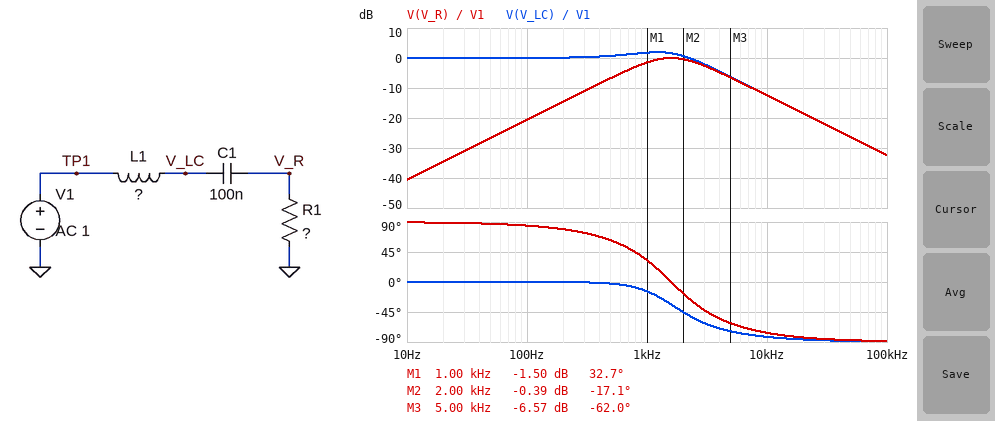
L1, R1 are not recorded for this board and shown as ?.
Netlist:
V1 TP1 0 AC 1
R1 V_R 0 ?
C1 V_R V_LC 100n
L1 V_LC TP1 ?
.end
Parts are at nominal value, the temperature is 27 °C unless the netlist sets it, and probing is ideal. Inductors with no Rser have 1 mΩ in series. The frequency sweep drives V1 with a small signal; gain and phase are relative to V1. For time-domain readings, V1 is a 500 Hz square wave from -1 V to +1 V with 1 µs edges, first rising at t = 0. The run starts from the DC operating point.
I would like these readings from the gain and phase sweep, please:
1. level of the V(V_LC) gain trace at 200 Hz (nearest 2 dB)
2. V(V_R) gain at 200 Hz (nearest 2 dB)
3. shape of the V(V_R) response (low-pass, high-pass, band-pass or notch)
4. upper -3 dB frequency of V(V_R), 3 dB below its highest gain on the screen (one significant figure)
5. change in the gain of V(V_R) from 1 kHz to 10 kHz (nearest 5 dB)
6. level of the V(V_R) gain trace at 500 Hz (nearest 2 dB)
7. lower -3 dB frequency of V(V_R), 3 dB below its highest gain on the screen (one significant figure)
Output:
0 dB
-14 dB
band-pass
3 kHz
-10 dB
-6 dB
800 Hz
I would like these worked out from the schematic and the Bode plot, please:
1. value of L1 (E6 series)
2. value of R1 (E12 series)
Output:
100 mH
1.5 kΩ
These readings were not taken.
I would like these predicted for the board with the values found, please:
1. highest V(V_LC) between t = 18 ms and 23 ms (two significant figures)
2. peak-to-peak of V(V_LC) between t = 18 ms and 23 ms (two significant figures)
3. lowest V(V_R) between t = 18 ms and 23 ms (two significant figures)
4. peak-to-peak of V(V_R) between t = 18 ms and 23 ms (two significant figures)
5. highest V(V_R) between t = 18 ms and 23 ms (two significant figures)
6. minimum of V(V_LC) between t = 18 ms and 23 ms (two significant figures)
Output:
1.4 V
2.8 V
-1.3 V
2.6 V
1.3 V
-1.4 V
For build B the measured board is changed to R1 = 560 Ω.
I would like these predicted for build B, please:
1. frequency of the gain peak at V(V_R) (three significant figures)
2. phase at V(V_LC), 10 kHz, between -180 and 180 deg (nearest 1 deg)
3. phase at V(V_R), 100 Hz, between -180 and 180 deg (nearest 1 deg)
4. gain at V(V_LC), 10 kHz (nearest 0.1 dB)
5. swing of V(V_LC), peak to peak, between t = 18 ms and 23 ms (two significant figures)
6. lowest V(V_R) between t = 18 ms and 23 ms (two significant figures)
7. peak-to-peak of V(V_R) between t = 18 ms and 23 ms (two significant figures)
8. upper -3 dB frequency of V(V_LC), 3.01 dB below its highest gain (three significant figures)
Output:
1.59 kHz
-101 deg
88 deg
-20.5 dB
4.0 V
-820 mV
1.6 V
1.92 kHz
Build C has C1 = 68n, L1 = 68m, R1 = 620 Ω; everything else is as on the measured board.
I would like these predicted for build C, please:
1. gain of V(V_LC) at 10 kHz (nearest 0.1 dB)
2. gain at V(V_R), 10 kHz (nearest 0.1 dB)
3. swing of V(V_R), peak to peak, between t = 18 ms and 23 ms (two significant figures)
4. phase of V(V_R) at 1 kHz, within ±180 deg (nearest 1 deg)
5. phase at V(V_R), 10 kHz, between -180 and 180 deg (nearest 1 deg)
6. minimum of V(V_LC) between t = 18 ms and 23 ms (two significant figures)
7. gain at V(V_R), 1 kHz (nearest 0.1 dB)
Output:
-15.8 dB
-16.4 dB
1.6 V
72 deg
-81 deg
-1.9 V
-10.2 dB
